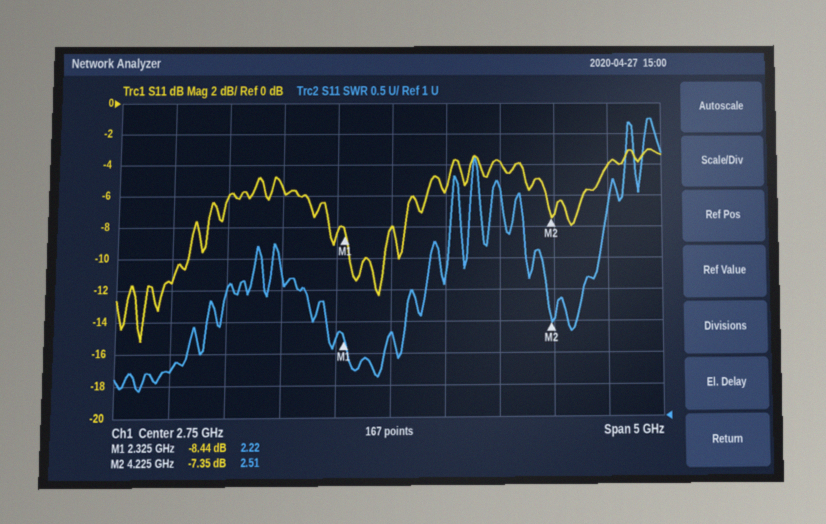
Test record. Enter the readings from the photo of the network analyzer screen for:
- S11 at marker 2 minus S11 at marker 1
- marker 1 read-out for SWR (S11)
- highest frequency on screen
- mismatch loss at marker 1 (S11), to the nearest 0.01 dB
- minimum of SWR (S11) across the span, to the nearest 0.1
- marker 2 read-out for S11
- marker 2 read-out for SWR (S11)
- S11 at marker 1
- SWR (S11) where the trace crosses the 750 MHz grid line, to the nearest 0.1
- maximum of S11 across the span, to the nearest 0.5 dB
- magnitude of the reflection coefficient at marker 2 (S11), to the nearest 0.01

1.09 dB
2.22
5.25 GHz
0.67 dB
1.4
-7.35 dB
2.51
-8.44 dB
1.7
-3.0 dB
0.43
